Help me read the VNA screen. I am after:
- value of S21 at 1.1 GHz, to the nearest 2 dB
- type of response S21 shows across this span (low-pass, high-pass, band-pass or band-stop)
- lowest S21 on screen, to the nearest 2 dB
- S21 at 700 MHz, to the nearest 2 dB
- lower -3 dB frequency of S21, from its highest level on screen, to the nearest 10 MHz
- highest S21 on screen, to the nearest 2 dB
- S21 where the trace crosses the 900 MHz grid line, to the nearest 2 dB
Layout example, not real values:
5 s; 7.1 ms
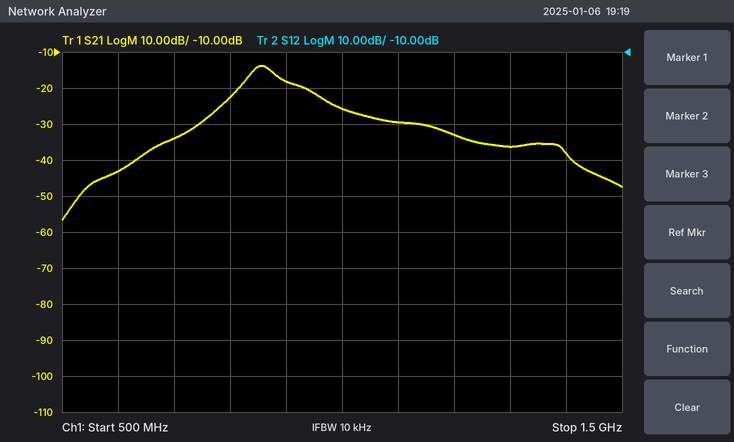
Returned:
-30 dB; band-pass; -56 dB; -34 dB; 830 MHz; -14 dB; -18 dB
